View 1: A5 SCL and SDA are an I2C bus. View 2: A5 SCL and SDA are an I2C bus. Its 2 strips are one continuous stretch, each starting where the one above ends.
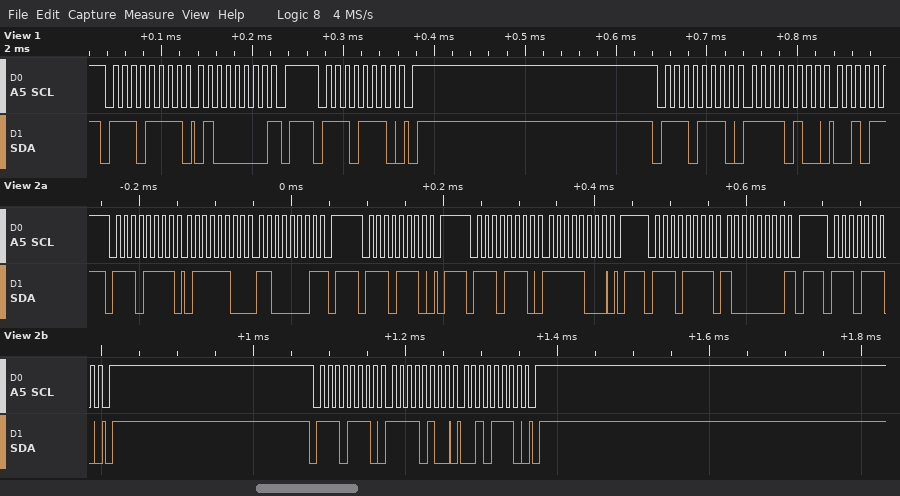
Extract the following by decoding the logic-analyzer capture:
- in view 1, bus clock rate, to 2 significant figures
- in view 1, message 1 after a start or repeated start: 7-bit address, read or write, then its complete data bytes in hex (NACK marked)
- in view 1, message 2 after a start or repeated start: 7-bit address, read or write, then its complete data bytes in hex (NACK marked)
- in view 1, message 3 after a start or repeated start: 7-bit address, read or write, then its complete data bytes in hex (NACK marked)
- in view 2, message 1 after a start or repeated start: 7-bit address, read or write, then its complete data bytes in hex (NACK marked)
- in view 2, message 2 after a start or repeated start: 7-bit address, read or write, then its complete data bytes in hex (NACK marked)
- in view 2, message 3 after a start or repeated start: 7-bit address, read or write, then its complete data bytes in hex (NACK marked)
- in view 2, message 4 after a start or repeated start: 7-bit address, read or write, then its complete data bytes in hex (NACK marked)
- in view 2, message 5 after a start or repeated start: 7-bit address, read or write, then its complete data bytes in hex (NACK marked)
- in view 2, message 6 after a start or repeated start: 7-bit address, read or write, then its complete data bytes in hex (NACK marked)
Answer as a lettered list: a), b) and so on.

a) 100 kHz
b) 0x77 read: 40 NACK
c) 0x77 write
d) 0x77 write: F4
e) 0x77 read: 7C C1 NACK
f) 0x77 write
g) 0x77 write: F8
h) 0x77 read: 80 NACK
i) 0x77 write
j) 0x77 write: F4 2E
